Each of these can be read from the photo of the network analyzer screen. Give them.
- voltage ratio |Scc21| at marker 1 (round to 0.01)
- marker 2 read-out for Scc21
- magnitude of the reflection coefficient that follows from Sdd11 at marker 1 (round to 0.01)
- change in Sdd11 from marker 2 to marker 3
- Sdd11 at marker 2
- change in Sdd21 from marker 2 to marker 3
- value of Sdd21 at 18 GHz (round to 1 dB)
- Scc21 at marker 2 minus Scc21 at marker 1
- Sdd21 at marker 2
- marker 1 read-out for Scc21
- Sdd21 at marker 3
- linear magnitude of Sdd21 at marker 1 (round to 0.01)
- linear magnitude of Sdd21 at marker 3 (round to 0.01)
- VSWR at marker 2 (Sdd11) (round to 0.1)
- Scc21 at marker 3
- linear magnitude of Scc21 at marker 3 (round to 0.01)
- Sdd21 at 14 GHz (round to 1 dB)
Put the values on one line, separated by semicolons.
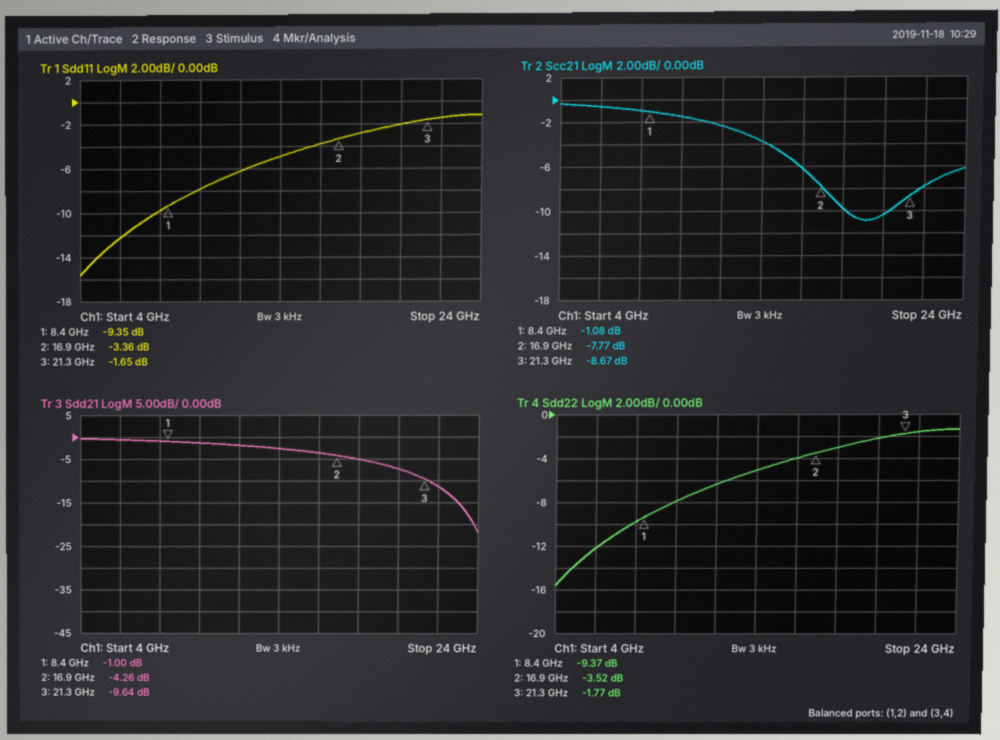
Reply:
0.88; -7.77 dB; 0.34; 1.71 dB; -3.36 dB; -5.38 dB; -5 dB; -6.69 dB; -4.26 dB; -1.08 dB; -9.64 dB; 0.89; 0.33; 5.2; -8.67 dB; 0.37; -3 dB
